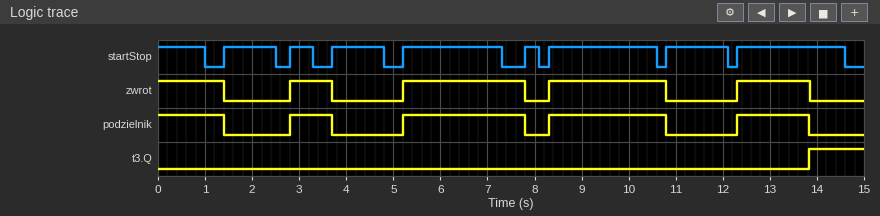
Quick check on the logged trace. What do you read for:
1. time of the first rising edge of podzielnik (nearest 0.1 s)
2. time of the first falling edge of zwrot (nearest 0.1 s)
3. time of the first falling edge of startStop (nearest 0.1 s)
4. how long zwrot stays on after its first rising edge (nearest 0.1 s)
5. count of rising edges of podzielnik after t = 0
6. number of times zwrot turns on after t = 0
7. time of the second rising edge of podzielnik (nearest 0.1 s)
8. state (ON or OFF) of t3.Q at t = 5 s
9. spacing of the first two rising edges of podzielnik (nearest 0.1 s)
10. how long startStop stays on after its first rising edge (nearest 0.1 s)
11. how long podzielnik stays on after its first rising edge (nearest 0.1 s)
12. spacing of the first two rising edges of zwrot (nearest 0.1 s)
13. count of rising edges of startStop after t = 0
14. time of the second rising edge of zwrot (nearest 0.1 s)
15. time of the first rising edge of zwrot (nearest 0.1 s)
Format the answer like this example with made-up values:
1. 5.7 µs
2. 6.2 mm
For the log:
1. 2.8 s
2. 1.4 s
3. 1.0 s
4. 0.9 s
5. 4
6. 4
7. 5.2 s
8. OFF
9. 2.4 s
10. 1.1 s
11. 0.9 s
12. 2.4 s
13. 8
14. 5.2 s
15. 2.8 s
